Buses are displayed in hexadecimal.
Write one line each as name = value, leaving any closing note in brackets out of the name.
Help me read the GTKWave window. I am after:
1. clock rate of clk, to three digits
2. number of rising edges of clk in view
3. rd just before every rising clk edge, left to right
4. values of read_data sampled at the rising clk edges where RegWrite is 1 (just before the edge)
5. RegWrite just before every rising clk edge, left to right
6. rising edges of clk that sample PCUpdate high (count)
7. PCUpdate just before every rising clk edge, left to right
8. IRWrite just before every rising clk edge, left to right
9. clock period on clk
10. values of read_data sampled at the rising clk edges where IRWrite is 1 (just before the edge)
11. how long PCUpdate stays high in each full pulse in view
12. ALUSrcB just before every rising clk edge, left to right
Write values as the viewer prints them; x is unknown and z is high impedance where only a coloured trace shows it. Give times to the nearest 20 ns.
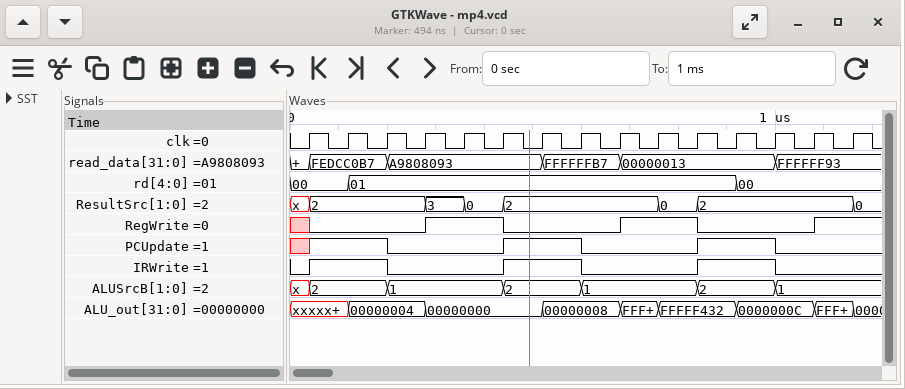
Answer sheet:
clock rate of clk, to three digits = 12.5 MHz
number of rising edges of clk in view = 15
rd just before every rising clk edge, left to right = 00, 00, 01, 01, 01, 01, 01, 01, 01, 01, 01, 01, 00, 00, 00
values of read_data sampled at the rising clk edges where RegWrite is 1 = A9808093, A9808093, 00000013, 00000013, FFFFFF93
RegWrite just before every rising clk edge, left to right = x 0 0 0 1 1 0 0 0 1 1 0 0 0 1
rising edges of clk that sample PCUpdate high = 6
PCUpdate just before every rising clk edge, left to right = x 1 1 0 0 0 1 1 0 0 0 1 1 0 0
IRWrite just before every rising clk edge, left to right = 0 1 1 0 0 0 1 1 0 0 0 1 1 0 0
clock period on clk = 80 ns
values of read_data sampled at the rising clk edges where IRWrite is 1 = FEDCC0B7, FEDCC0B7, A9808093, FFFFFFB7, 00000013, 00000013
how long PCUpdate stays high in each full pulse in view = 160 ns, 160 ns
ALUSrcB just before every rising clk edge, left to right = x, 2, 2, 1, 1, 1, 2, 2, 1, 1, 1, 2, 2, 1, 1
